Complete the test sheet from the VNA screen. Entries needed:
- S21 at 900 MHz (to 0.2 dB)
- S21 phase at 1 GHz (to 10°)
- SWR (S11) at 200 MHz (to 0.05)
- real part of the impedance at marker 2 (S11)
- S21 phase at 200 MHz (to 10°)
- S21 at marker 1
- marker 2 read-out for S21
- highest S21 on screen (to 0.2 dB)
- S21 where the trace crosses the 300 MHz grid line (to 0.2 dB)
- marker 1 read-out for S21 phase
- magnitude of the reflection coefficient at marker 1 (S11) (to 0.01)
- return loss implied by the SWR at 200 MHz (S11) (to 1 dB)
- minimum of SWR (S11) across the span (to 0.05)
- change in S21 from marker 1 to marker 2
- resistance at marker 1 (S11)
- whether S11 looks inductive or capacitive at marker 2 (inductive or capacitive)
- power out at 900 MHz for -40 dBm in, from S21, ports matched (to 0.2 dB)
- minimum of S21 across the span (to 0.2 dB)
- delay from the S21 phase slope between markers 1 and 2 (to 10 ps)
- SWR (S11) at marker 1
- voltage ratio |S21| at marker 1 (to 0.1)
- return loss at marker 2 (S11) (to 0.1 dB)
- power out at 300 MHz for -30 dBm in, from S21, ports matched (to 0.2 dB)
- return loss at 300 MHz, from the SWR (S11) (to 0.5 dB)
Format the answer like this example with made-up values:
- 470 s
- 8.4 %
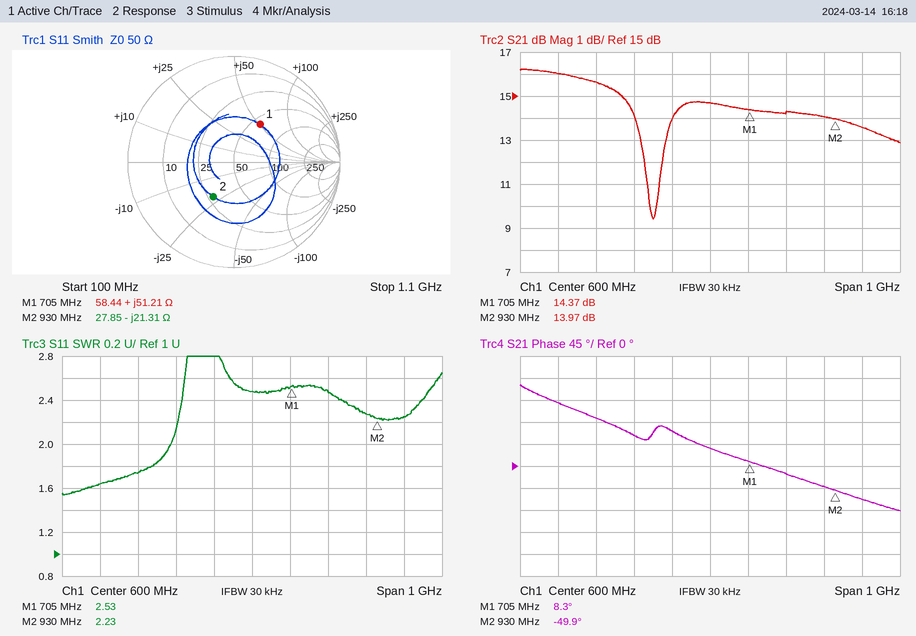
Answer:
- 14.0 dB
- -70°
- 1.65
- 27.85 Ω
- 130°
- 14.37 dB
- 13.97 dB
- 16.2 dB
- 15.6 dB
- 8.3°
- 0.43
- 12 dB
- 1.55
- -0.40 dB
- 58.44 Ω
- capacitive
- -26.0 dBm
- 9.4 dB
- 720 ps
- 2.53
- 5.2
- 8.4 dB
- -14.4 dBm
- 11.5 dB
